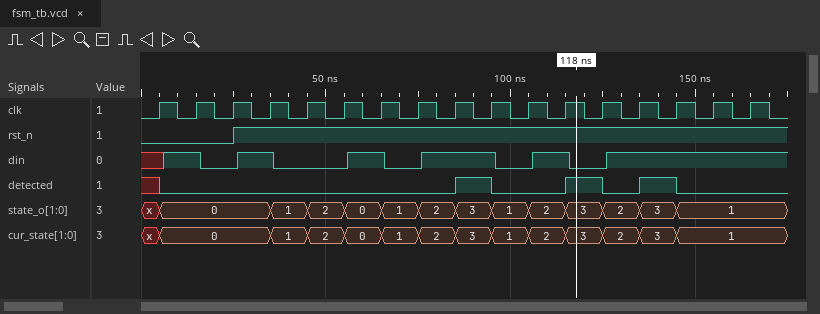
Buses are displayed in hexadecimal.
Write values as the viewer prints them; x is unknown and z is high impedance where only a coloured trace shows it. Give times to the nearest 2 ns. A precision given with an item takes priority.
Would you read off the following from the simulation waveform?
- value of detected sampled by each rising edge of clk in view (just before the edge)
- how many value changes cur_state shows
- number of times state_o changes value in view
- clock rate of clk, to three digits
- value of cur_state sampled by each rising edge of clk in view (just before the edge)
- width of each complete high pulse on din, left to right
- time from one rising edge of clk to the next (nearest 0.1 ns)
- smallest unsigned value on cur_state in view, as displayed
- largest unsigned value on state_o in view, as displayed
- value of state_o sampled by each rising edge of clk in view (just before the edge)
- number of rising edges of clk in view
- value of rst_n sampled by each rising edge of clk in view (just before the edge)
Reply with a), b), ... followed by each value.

a) x 0 0 0 0 0 0 0 0 1 0 0 1 0 1 0 0
b) 13
c) 13
d) 100 MHz
e) x, 0, 0, 0, 1, 2, 0, 1, 2, 3, 1, 2, 3, 2, 3, 1, 1
f) 10 ns, 10 ns, 20 ns, 10 ns
g) 10 ns
h) 0
i) 3
j) x, 0, 0, 0, 1, 2, 0, 1, 2, 3, 1, 2, 3, 2, 3, 1, 1
k) 17
l) 0 0 0 1 1 1 1 1 1 1 1 1 1 1 1 1 1
